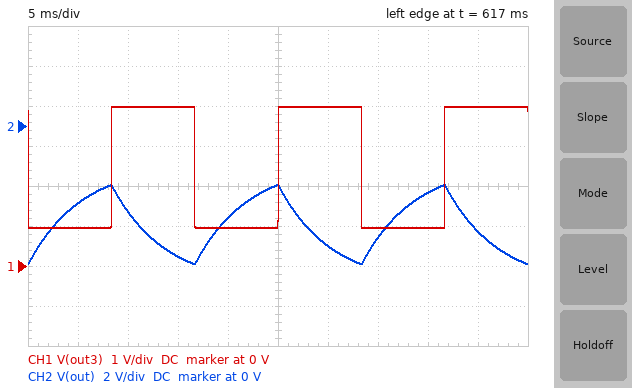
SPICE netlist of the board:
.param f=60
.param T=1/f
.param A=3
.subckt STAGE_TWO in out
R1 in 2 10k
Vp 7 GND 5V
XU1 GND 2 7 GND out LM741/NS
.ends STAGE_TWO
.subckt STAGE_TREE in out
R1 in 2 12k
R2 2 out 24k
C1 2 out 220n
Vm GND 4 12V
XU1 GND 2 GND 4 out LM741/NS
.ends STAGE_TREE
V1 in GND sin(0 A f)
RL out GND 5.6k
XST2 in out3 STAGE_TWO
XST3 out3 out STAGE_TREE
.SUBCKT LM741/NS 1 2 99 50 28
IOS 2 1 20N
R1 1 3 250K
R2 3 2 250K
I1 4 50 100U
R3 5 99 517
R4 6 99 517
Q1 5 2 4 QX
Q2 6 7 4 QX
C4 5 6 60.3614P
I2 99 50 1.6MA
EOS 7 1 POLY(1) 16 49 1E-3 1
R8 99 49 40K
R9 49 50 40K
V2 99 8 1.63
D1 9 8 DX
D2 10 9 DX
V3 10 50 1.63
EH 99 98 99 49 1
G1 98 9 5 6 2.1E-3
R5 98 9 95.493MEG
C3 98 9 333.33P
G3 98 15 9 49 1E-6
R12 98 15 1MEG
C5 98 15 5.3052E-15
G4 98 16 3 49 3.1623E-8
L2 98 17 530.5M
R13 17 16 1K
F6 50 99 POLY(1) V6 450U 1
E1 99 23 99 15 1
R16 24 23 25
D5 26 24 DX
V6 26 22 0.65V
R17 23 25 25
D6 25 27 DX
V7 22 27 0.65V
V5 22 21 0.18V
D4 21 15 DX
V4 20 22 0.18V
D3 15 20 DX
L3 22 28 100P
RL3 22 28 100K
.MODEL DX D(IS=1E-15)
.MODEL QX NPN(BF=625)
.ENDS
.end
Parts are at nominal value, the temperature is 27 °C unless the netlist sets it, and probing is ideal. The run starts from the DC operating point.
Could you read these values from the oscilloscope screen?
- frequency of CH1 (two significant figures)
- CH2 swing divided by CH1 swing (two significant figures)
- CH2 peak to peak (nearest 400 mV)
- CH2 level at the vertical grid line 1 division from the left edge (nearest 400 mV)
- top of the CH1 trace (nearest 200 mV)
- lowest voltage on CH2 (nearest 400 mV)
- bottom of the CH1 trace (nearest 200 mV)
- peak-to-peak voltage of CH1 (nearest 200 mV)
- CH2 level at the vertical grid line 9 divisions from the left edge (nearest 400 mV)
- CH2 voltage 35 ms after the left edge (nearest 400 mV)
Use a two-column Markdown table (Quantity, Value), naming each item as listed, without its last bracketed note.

| Quantity | Value |
|---|---|
| frequency of CH1 | 60 Hz |
| CH2 swing divided by CH1 swing | 1.3 |
| CH2 peak to peak | 4.0 V |
| CH2 level at the vertical grid line 1 division from the left edge | -4.0 V |
| top of the CH1 trace | 4.0 V |
| lowest voltage on CH2 | -6.8 V |
| bottom of the CH1 trace | 1.0 V |
| peak-to-peak voltage of CH1 | 3.0 V |
| CH2 level at the vertical grid line 9 divisions from the left edge | -5.2 V |
| CH2 voltage 35 ms after the left edge | -5.6 V |
